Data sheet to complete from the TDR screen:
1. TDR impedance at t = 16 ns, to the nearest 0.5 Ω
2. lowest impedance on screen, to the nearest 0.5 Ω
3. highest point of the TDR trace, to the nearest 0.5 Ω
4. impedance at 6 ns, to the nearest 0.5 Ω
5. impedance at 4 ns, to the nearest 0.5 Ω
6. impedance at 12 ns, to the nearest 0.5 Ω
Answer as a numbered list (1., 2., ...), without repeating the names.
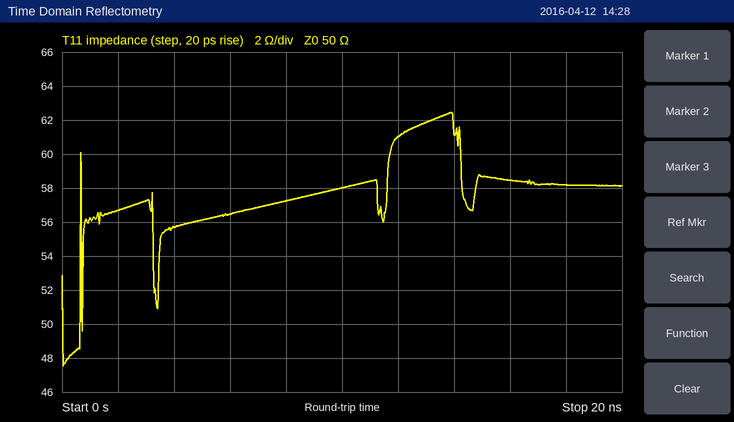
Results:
1. 58.5 Ω
2. 47.5 Ω
3. 62.5 Ω
4. 56.5 Ω
5. 55.5 Ω
6. 61.0 Ω
